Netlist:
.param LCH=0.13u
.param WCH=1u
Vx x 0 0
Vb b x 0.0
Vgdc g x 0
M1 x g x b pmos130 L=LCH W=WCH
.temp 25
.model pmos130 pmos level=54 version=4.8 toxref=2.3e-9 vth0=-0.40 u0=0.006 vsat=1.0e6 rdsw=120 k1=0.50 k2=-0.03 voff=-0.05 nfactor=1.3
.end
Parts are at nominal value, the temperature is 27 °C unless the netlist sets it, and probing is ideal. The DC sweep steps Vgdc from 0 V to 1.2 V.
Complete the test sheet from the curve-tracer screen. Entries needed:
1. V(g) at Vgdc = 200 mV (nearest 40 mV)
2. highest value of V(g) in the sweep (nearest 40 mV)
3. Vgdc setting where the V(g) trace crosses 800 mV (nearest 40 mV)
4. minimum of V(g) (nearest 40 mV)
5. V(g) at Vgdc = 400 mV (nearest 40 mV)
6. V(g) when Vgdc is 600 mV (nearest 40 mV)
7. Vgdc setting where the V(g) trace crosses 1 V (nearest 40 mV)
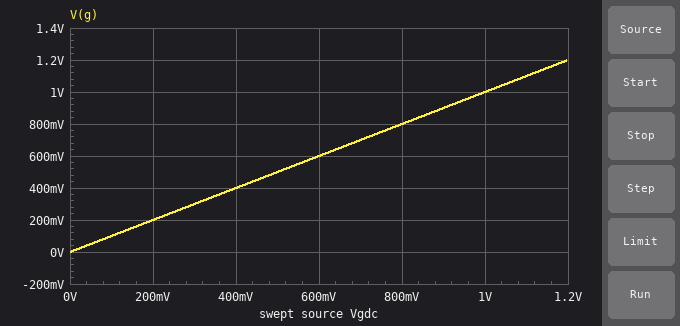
200 mV
1.20 V
800 mV
0 V
400 mV
600 mV
1.00 V
